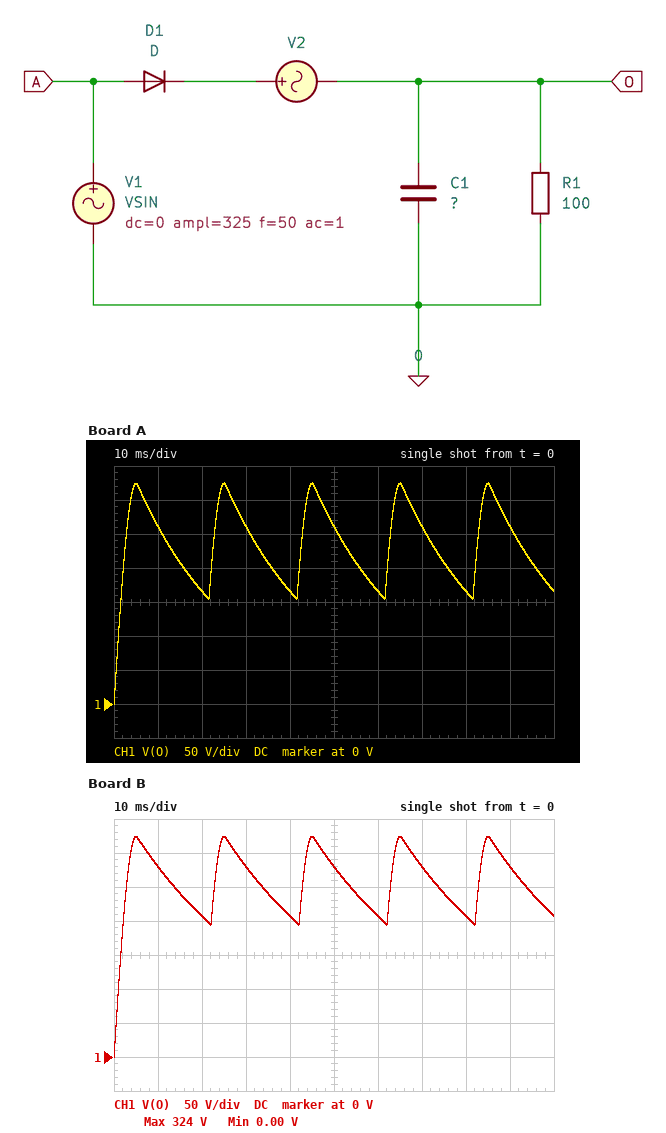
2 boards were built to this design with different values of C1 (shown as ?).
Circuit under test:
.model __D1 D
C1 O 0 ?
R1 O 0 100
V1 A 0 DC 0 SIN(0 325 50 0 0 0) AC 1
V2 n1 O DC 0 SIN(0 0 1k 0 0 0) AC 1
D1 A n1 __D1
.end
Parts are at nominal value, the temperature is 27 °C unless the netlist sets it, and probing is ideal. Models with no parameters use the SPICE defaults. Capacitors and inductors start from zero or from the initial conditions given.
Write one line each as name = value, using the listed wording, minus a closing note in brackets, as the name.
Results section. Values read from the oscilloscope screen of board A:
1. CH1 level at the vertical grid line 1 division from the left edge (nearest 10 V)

CH1 level at the vertical grid line 1 division from the left edge = 260 V
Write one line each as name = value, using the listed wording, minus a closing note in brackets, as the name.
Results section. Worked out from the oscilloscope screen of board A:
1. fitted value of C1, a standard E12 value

fitted value of C1, a standard E12 value = 220 µF
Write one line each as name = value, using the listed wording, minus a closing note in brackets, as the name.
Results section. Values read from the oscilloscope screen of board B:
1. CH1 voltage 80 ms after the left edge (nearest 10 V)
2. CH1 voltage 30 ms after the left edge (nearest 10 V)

CH1 voltage 80 ms after the left edge = 210 V
CH1 voltage 30 ms after the left edge = 280 V
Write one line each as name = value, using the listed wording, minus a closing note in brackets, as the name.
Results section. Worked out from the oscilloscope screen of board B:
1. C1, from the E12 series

C1, from the E12 series = 330 µF
